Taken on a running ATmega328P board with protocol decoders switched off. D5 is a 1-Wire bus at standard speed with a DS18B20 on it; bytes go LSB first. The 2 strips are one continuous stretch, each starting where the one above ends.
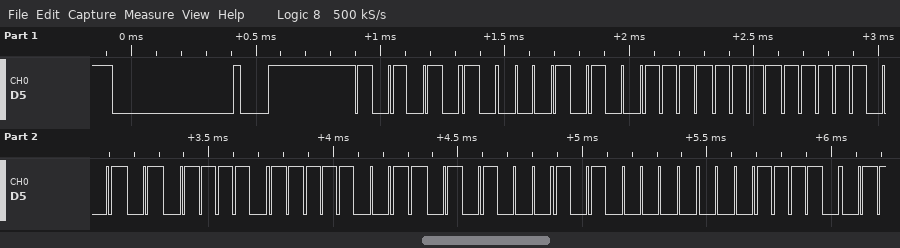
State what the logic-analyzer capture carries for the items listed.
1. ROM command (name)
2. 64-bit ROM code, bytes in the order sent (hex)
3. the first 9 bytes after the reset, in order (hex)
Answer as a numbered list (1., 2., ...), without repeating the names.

1. Match ROM
2. 28 FF 9F 7A 9F 15 05 78
3. 55 28 FF 9F 7A 9F 15 05 78
